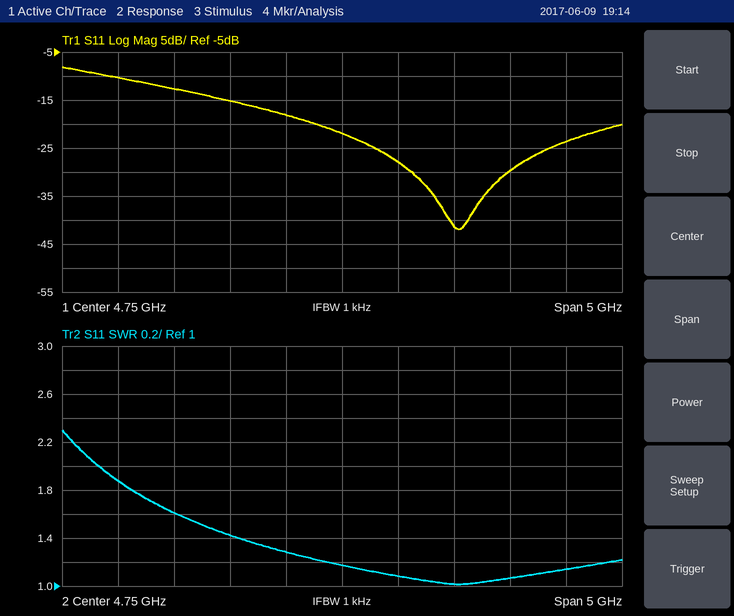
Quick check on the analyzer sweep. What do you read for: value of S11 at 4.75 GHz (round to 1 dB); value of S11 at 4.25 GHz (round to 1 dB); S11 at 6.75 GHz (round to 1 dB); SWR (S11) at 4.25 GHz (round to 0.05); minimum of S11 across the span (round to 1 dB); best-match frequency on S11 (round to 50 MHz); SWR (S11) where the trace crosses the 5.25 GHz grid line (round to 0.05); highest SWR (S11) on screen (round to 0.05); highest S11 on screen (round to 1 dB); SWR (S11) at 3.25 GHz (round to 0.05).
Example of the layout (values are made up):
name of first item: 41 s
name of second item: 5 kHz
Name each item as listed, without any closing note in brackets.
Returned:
value of S11 at 4.75 GHz: -22 dB
value of S11 at 4.25 GHz: -18 dB
S11 at 6.75 GHz: -24 dB
SWR (S11) at 4.25 GHz: 1.30
minimum of S11 across the span: -42 dB
best-match frequency on S11: 5.80 GHz
SWR (S11) where the trace crosses the 5.25 GHz grid line: 1.10
highest SWR (S11) on screen: 2.30
highest S11 on screen: -8 dB
SWR (S11) at 3.25 GHz: 1.60
